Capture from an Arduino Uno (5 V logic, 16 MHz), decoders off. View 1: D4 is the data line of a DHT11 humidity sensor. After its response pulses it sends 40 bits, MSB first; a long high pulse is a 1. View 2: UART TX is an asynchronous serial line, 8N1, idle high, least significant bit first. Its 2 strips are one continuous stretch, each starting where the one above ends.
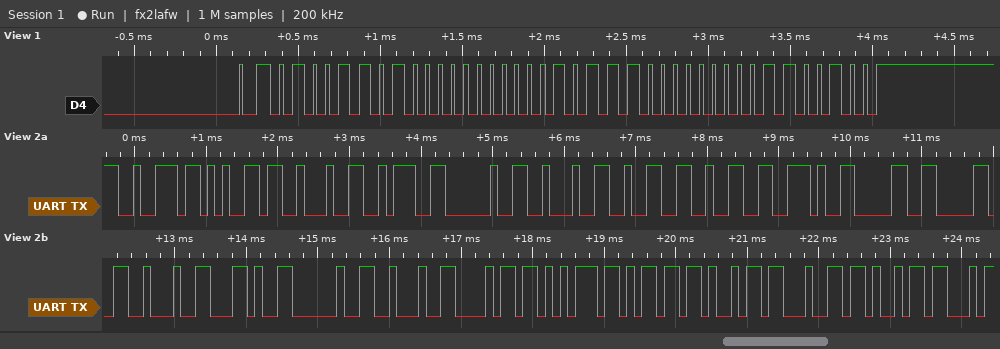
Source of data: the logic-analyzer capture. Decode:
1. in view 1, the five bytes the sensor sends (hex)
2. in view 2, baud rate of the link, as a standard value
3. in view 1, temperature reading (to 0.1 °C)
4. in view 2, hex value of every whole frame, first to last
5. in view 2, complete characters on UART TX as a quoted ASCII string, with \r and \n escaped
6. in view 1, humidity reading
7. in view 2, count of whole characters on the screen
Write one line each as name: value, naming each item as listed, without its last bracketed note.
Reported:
in view 1, the five bytes the sensor sends: 4D 00 17 00 64
in view 2, baud rate of the link, as a standard value: 9600 baud
in view 1, temperature reading: 23.0 °C
in view 2, hex value of every whole frame, first to last: 72 65 22 3A 20 22 32 32 2E 30 30 22 2C 20 22 68 75 6D 69 64 69
in view 2, complete characters on UART TX as a quoted ASCII string, with \r and \n escaped: "re\": \"22.00\", \"humidi"
in view 1, humidity reading: 77 %
in view 2, count of whole characters on the screen: 21
